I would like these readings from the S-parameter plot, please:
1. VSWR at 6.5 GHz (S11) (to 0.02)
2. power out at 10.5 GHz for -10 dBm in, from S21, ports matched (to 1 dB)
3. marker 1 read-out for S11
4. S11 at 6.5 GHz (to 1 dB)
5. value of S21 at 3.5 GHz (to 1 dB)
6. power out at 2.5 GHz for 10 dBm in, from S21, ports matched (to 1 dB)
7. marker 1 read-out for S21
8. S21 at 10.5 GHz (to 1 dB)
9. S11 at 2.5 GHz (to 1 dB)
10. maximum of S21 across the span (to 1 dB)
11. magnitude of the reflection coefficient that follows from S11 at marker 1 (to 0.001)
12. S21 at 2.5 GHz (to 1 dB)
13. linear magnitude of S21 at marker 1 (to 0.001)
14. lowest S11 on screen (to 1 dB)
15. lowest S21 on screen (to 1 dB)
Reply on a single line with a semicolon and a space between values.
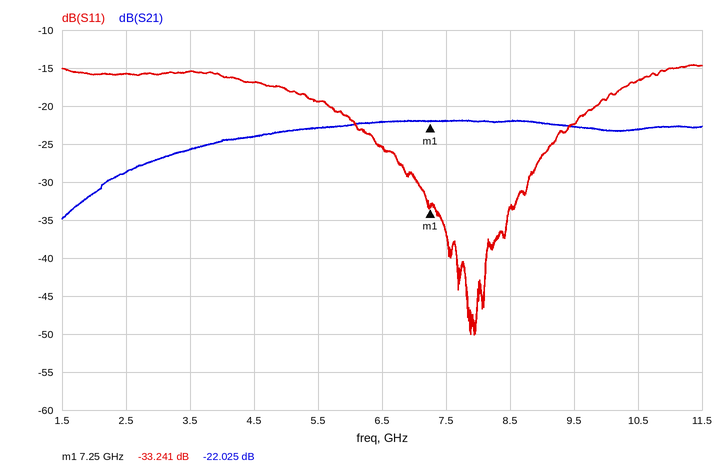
1.12; -33 dBm; -33.241 dB; -25 dB; -26 dB; -19 dBm; -22.025 dB; -23 dB; -16 dB; -22 dB; 0.022; -29 dB; 0.079; -50 dB; -35 dB
